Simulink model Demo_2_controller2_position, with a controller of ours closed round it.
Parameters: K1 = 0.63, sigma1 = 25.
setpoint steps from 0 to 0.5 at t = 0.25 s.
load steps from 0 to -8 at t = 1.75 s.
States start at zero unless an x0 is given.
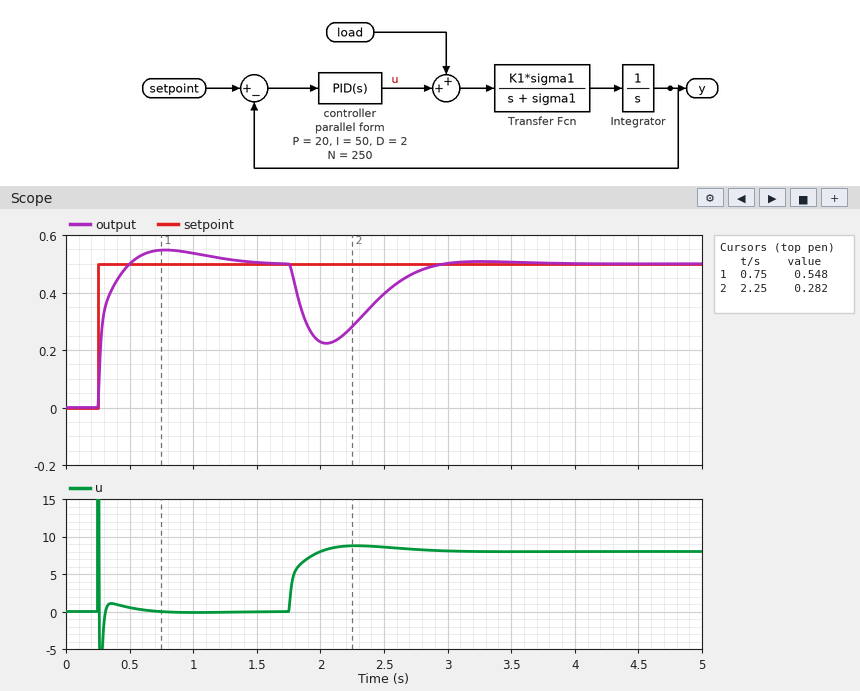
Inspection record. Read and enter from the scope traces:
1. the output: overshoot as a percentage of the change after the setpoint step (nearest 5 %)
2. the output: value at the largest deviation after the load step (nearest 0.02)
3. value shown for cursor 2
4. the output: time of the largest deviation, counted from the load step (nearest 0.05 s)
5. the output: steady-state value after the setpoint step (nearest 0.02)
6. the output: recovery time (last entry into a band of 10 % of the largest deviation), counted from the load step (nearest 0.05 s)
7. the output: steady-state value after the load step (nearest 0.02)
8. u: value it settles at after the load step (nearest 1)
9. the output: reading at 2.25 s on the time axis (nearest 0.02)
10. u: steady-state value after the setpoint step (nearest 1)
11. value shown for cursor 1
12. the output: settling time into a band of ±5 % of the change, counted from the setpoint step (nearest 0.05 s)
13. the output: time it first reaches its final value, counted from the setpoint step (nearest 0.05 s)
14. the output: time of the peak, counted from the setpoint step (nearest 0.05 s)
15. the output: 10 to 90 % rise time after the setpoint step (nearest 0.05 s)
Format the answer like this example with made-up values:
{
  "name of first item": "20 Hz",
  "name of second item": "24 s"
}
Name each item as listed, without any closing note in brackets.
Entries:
{
  "the output: overshoot as a percentage of the change after the setpoint step": "10 %",
  "the output: value at the largest deviation after the load step": "0.22",
  "value shown for cursor 2": "0.282",
  "the output: time of the largest deviation, counted from the load step": "0.30 s",
  "the output: steady-state value after the setpoint step": "0.50",
  "the output: recovery time (last entry into a band of 10 % of the largest deviation), counted from the load step": "1.00 s",
  "the output: steady-state value after the load step": "0.50",
  "u: value it settles at after the load step": "8",
  "the output: reading at 2.25 s on the time axis": "0.28",
  "u: steady-state value after the setpoint step": "0",
  "value shown for cursor 1": "0.548",
  "the output: settling time into a band of ±5 % of the change, counted from the setpoint step": "0.90 s",
  "the output: time it first reaches its final value, counted from the setpoint step": "0.25 s",
  "the output: time of the peak, counted from the setpoint step": "0.55 s",
  "the output: 10 to 90 % rise time after the setpoint step": "0.15 s"
}
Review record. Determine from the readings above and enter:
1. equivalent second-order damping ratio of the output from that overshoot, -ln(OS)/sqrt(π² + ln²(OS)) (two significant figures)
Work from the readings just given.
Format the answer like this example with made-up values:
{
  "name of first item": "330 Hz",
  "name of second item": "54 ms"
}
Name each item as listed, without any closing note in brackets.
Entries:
{
  "equivalent second-order damping ratio of the output from that overshoot, -ln(OS)/sqrt(π² + ln²(OS))": "0.59"
}
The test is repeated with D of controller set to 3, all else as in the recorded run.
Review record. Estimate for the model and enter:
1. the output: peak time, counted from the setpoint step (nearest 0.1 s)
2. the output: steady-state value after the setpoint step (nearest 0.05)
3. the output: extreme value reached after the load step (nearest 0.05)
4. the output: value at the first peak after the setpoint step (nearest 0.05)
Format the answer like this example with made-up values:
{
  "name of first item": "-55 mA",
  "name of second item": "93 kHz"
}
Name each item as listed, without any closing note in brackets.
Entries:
{
  "the output: peak time, counted from the setpoint step": "0.6 s",
  "the output: steady-state value after the setpoint step": "0.50",
  "the output: extreme value reached after the load step": "0.25",
  "the output: value at the first peak after the setpoint step": "0.55"
}
